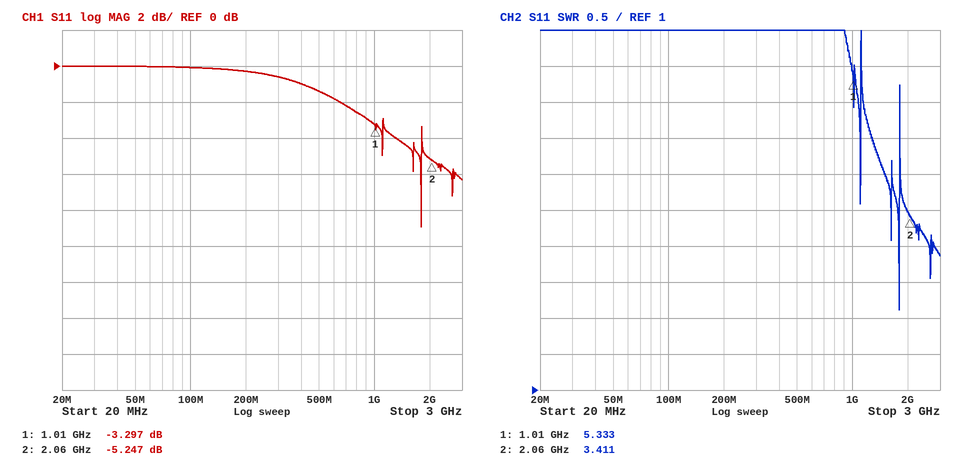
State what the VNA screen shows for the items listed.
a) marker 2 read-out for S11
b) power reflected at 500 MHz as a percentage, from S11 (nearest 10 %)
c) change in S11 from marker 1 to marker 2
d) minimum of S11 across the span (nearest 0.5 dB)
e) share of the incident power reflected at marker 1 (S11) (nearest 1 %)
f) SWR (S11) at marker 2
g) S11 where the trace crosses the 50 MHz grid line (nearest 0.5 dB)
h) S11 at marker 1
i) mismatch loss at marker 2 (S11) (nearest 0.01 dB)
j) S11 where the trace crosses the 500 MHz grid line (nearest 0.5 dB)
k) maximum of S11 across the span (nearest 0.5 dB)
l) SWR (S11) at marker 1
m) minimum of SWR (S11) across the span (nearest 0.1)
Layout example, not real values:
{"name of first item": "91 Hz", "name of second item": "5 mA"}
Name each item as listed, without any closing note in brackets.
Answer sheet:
{"marker 2 read-out for S11": "-5.247 dB", "power reflected at 500 MHz as a percentage, from S11": "70 %", "change in S11 from marker 1 to marker 2": "-1.950 dB", "minimum of S11 across the span": "-9.0 dB", "share of the incident power reflected at marker 1 (S11)": "47 %", "SWR (S11) at marker 2": "3.411", "S11 where the trace crosses the 50 MHz grid line": "0.0 dB", "S11 at marker 1": "-3.297 dB", "mismatch loss at marker 2 (S11)": "1.54 dB", "S11 where the trace crosses the 500 MHz grid line": "-1.5 dB", "maximum of S11 across the span": "0.0 dB", "SWR (S11) at marker 1": "5.333", "minimum of SWR (S11) across the span": "2.1"}
